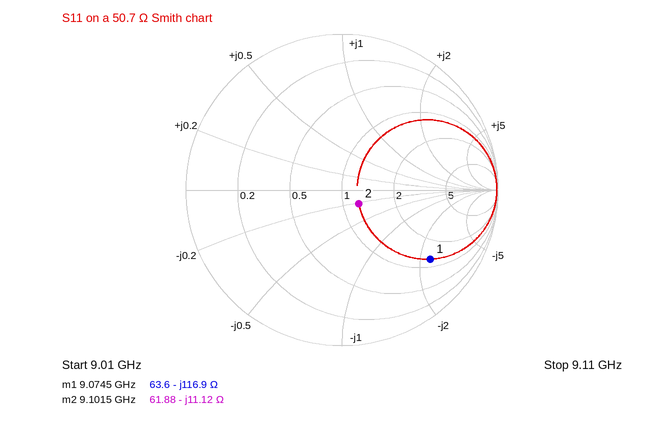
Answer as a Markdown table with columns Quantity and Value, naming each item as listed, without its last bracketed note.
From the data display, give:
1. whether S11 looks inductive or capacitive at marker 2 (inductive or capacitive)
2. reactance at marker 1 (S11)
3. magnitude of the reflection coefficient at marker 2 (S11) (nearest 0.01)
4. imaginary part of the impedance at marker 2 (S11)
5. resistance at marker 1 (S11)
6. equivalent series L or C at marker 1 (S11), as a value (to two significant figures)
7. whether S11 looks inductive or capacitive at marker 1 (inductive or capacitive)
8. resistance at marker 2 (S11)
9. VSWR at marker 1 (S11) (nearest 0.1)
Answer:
| Quantity | Value |
|---|---|
| whether S11 looks inductive or capacitive at marker 2 | capacitive |
| reactance at marker 1 | -116.9 Ω |
| magnitude of the reflection coefficient at marker 2 (S11) | 0.14 |
| imaginary part of the impedance at marker 2 | -11.12 Ω |
| resistance at marker 1 | 63.6 Ω |
| equivalent series L or C at marker 1 (S11), as a value | 150 fF |
| whether S11 looks inductive or capacitive at marker 1 | capacitive |
| resistance at marker 2 | 61.88 Ω |
| VSWR at marker 1 (S11) | 6.1 |
